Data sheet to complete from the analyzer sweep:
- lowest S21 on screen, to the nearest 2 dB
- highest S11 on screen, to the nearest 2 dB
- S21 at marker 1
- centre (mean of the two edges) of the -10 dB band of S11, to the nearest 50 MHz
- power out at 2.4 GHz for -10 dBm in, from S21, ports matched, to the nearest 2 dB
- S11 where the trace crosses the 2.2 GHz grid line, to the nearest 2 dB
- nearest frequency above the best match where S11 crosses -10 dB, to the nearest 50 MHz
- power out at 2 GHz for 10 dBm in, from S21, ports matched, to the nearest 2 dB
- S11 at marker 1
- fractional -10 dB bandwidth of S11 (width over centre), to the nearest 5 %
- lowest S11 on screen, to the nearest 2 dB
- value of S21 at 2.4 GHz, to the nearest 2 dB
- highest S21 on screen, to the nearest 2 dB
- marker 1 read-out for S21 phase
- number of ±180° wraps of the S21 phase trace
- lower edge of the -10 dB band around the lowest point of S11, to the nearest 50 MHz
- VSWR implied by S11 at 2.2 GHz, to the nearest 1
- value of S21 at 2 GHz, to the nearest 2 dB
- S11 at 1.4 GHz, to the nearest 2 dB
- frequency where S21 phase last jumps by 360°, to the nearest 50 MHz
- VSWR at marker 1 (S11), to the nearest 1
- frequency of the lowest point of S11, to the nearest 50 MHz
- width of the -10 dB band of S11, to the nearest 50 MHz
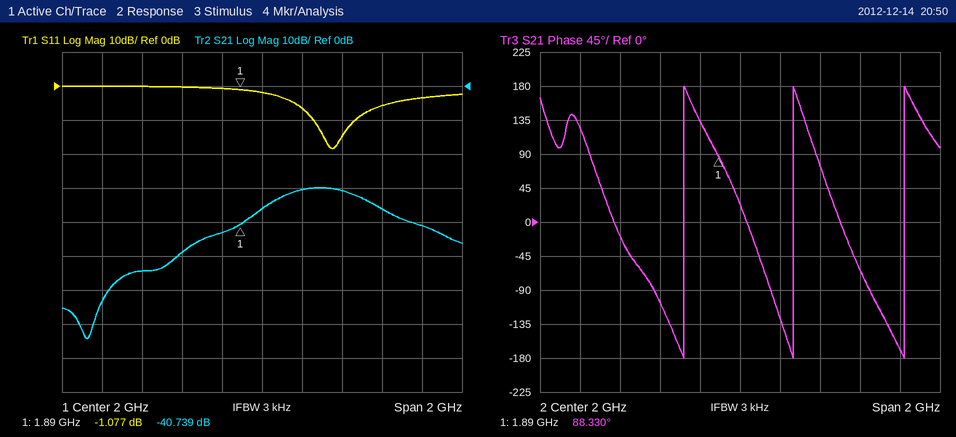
-74 dB
0 dB
-40.739 dB
2.35 GHz
-40 dBm
-6 dB
2.45 GHz
-26 dBm
-1.077 dB
10 %
-18 dB
-30 dB
-30 dB
88.330°
3
2.25 GHz
3
-36 dB
0 dB
2.80 GHz
16
2.35 GHz
200 MHz
